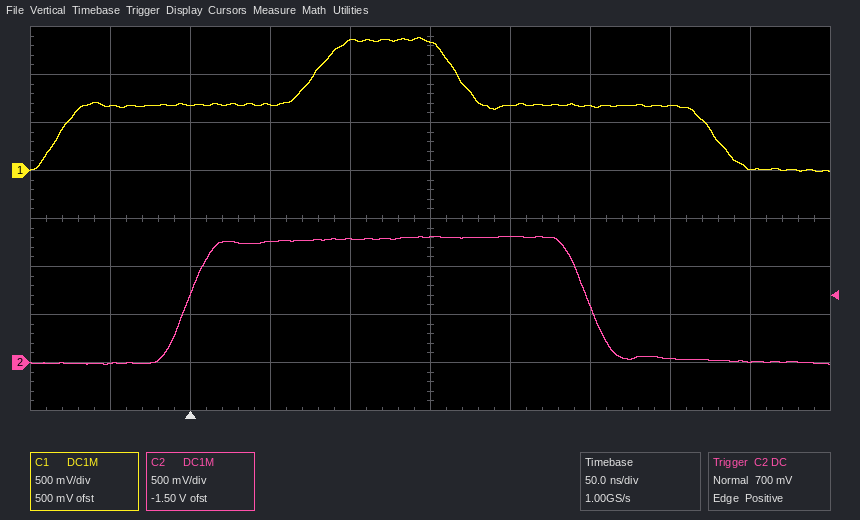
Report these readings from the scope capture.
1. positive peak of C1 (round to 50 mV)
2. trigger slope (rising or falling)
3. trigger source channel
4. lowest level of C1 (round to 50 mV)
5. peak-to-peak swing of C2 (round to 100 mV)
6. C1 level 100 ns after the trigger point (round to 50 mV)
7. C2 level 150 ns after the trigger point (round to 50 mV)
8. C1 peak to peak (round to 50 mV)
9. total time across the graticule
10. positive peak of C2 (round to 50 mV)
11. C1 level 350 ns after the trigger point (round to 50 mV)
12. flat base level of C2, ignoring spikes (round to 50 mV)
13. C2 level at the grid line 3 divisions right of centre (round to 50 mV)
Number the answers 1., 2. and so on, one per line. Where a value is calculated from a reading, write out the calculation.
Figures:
1. 1.40 V
2. rising
3. C2
4. 0 mV
5. 1.30 V
6. 1.35 V
7. 1.30 V
8. 1.40 V − (0 mV) = 1.40 V
9. 500 ns
10. 1.30 V
11. 0 mV
12. 0 mV
13. 50 mV
